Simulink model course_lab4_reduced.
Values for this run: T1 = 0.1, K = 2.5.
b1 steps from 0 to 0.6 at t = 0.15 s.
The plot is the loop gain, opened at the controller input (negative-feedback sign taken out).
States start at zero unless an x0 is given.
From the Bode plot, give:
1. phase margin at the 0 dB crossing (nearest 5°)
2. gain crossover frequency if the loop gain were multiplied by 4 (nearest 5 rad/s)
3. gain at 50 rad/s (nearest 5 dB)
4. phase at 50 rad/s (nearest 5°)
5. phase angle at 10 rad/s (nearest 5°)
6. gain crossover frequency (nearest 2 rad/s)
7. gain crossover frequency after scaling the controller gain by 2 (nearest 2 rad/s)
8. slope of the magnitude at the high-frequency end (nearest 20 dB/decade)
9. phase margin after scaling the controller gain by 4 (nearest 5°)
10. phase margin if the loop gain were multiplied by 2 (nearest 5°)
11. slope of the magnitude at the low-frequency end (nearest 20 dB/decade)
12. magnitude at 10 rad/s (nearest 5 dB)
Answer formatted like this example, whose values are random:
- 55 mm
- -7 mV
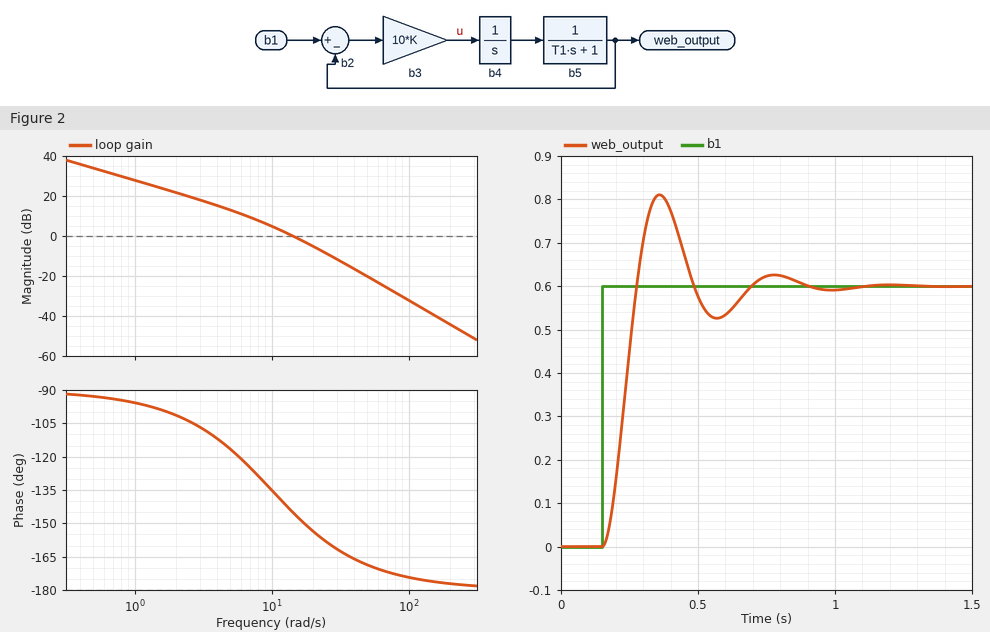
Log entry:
- 35°
- 30 rad/s
- -20 dB
- -170°
- -135°
- 14 rad/s
- 22 rad/s
- -40 dB/decade
- 20°
- 25°
- -20 dB/decade
- 5 dB
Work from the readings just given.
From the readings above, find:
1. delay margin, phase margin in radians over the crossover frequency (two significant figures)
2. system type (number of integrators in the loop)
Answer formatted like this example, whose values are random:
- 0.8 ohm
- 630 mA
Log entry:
- 0.044 s
- 1
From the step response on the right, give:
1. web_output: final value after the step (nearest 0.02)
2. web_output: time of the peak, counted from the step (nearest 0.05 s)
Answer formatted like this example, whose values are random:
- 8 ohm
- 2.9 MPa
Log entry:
- 0.60
- 0.20 s
